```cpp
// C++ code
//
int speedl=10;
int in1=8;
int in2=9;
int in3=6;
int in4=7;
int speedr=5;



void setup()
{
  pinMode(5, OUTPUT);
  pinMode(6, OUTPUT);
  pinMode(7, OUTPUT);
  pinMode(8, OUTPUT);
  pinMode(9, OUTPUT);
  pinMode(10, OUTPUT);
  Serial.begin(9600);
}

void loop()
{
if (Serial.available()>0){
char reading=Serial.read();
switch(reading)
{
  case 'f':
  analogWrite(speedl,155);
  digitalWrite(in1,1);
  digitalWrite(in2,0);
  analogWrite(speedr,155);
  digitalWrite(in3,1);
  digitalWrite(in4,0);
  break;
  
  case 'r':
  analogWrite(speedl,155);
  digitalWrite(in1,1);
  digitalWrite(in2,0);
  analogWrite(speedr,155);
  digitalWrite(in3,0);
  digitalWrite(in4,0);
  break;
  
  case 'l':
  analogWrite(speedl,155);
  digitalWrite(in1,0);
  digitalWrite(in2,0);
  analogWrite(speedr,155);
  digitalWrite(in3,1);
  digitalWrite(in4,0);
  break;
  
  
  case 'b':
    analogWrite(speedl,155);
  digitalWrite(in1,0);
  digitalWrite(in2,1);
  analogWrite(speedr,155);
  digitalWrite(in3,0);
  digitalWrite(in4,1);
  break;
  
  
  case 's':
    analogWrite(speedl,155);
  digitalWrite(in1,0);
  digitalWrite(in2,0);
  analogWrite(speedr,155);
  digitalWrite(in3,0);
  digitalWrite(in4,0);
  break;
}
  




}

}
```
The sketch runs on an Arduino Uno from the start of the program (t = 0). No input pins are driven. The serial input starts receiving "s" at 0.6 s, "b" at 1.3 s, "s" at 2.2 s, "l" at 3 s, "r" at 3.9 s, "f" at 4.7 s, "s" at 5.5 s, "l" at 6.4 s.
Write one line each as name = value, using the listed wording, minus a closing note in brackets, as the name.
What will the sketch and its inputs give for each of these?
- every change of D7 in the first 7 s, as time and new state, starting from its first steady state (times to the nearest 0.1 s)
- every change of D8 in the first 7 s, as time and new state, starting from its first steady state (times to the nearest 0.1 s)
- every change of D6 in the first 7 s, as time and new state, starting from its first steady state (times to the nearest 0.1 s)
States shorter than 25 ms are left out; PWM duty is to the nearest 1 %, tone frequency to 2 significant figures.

every change of D7 in the first 7 s, as time and new state, starting from its first steady state = 0 s low; 1.3 s high; 2.2 s low
every change of D8 in the first 7 s, as time and new state, starting from its first steady state = 0 s low; 3.9 s high; 5.5 s low
every change of D6 in the first 7 s, as time and new state, starting from its first steady state = 0 s low; 3 s high; 3.9 s low; 4.7 s high; 5.5 s low; 6.4 s high
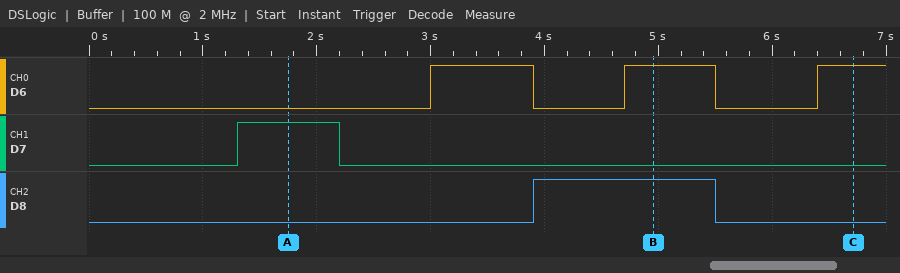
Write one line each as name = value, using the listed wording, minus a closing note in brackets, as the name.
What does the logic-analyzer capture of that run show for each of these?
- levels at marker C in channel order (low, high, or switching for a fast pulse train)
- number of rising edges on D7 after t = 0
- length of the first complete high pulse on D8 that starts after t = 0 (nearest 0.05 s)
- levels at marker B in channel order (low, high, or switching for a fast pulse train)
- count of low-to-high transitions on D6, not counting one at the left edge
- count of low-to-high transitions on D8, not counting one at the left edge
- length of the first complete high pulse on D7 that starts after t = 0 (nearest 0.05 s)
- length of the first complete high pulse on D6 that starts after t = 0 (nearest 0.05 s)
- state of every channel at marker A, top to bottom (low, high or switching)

levels at marker C in channel order = D6 high, D7 low, D8 low
number of rising edges on D7 after t = 0 = 1
length of the first complete high pulse on D8 that starts after t = 0 = 1.60 s
levels at marker B in channel order = D6 high, D7 low, D8 high
count of low-to-high transitions on D6, not counting one at the left edge = 3
count of low-to-high transitions on D8, not counting one at the left edge = 1
length of the first complete high pulse on D7 that starts after t = 0 = 0.90 s
length of the first complete high pulse on D6 that starts after t = 0 = 0.90 s
state of every channel at marker A, top to bottom = D6 low, D7 high, D8 low
